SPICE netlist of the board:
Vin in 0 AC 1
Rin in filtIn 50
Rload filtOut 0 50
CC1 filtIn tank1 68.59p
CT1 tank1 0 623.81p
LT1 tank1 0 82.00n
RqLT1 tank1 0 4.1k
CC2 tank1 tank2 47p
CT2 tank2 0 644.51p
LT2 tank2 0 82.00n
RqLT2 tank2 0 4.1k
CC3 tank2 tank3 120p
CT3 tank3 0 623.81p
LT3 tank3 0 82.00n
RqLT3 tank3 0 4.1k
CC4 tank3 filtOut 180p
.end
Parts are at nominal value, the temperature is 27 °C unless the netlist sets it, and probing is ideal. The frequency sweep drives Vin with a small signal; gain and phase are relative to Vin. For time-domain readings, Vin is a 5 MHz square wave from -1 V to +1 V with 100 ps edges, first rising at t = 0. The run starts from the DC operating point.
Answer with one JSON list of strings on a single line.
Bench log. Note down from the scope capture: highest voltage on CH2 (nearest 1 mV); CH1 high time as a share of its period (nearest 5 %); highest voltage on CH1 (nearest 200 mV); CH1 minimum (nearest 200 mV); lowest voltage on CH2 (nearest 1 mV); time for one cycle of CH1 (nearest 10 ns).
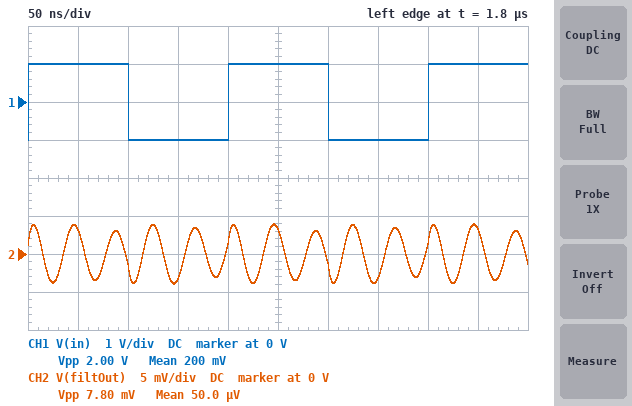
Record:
["4 mV", "50 %", "1.0 V", "-1.0 V", "-4 mV", "200 ns"]
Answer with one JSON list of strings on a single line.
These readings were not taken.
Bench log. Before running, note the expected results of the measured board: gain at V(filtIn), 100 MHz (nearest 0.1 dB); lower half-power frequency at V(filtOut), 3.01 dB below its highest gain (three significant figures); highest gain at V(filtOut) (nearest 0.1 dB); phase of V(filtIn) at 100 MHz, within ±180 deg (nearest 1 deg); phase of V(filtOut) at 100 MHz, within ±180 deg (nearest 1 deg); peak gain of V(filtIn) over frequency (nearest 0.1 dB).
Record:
["-6.8 dB", "20.0 MHz", "-6.5 dB", "-63 deg", "-50 deg", "0 dB"]
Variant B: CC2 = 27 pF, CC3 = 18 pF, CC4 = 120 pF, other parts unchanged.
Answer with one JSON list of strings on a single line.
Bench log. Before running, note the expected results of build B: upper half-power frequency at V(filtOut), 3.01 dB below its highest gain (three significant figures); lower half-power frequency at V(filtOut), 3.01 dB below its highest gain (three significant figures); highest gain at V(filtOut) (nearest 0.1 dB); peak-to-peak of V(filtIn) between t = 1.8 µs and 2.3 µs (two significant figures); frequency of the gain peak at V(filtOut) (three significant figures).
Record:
["21.6 MHz", "20.6 MHz", "-8.7 dB", "2.1 V", "21.4 MHz"]
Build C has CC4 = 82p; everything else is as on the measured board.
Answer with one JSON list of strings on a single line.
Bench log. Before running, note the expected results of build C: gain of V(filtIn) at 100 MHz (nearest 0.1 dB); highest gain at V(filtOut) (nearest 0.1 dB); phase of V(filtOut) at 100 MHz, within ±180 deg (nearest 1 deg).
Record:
["-6.8 dB", "-7.1 dB", "-39 deg"]
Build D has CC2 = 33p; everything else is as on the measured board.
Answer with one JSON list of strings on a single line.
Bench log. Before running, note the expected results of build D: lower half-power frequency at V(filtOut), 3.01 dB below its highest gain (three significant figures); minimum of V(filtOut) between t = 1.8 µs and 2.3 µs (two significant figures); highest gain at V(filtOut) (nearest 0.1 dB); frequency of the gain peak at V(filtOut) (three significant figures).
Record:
["20.3 MHz", "-3.0 mV", "-6.9 dB", "20.9 MHz"]
